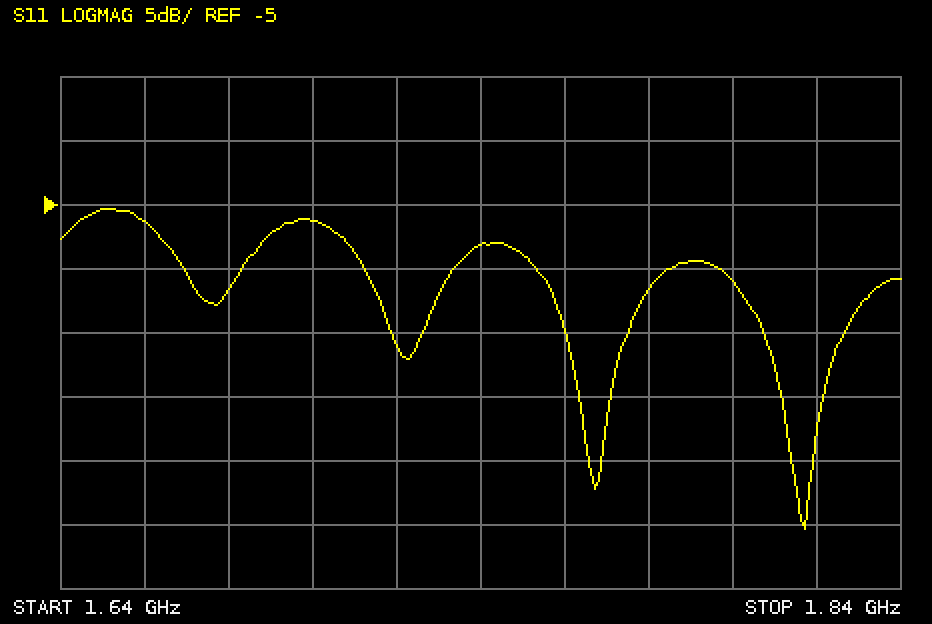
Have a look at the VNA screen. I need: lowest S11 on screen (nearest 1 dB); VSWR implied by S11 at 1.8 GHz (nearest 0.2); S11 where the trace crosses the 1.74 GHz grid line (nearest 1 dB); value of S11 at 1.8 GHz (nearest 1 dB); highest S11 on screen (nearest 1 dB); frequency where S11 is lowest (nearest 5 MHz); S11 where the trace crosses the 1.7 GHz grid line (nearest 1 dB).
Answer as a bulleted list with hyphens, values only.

- -30 dB
- 1.8
- -8 dB
- -11 dB
- -5 dB
- 1.815 GHz
- -6 dB
